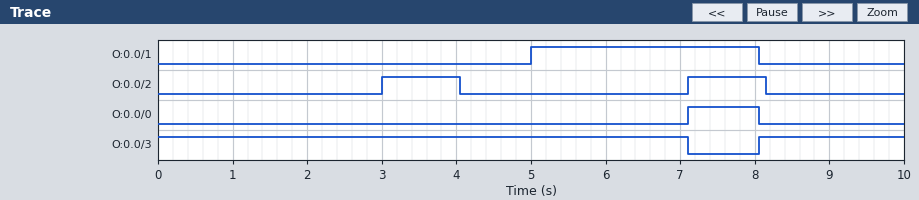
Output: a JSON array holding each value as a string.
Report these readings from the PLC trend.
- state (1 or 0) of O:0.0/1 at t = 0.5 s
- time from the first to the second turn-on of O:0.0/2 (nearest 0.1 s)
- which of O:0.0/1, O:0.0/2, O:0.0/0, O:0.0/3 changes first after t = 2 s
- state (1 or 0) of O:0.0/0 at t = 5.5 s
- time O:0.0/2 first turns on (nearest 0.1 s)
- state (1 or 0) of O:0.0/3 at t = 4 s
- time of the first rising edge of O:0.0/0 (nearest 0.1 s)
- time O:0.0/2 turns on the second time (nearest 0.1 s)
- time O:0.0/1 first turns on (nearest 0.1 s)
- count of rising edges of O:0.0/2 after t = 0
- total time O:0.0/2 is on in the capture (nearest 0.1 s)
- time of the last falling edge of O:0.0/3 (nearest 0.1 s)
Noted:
["0", "4.1 s", "O:0.0/2", "0", "3.0 s", "1", "7.1 s", "7.1 s", "5.0 s", "2", "2.1 s", "7.1 s"]
